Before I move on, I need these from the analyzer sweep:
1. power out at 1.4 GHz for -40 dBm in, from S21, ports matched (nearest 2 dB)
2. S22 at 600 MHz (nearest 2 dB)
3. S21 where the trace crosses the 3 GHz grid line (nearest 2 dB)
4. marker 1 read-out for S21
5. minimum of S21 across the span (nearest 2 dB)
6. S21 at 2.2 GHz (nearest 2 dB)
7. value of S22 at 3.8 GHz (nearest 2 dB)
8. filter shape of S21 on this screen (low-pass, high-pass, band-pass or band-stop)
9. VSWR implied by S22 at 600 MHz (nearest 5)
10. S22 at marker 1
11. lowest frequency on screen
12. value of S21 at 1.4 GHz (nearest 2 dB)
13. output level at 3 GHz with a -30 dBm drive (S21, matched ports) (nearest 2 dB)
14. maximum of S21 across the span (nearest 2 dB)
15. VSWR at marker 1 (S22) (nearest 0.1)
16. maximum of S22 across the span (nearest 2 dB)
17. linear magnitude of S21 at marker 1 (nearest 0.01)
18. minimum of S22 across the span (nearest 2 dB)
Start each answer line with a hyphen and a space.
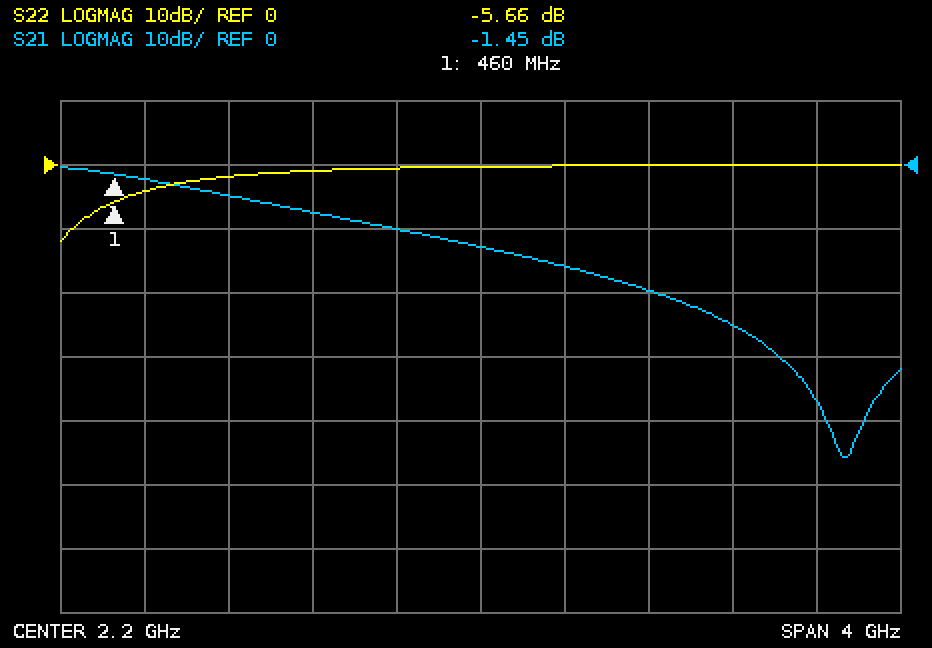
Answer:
- -48 dBm
- -4 dB
- -20 dB
- -1.45 dB
- -46 dB
- -12 dB
- 0 dB
- low-pass
- 5
- -5.66 dB
- 200 MHz
- -8 dB
- -50 dBm
- 0 dB
- 3.2
- 0 dB
- 0.85
- -12 dB
